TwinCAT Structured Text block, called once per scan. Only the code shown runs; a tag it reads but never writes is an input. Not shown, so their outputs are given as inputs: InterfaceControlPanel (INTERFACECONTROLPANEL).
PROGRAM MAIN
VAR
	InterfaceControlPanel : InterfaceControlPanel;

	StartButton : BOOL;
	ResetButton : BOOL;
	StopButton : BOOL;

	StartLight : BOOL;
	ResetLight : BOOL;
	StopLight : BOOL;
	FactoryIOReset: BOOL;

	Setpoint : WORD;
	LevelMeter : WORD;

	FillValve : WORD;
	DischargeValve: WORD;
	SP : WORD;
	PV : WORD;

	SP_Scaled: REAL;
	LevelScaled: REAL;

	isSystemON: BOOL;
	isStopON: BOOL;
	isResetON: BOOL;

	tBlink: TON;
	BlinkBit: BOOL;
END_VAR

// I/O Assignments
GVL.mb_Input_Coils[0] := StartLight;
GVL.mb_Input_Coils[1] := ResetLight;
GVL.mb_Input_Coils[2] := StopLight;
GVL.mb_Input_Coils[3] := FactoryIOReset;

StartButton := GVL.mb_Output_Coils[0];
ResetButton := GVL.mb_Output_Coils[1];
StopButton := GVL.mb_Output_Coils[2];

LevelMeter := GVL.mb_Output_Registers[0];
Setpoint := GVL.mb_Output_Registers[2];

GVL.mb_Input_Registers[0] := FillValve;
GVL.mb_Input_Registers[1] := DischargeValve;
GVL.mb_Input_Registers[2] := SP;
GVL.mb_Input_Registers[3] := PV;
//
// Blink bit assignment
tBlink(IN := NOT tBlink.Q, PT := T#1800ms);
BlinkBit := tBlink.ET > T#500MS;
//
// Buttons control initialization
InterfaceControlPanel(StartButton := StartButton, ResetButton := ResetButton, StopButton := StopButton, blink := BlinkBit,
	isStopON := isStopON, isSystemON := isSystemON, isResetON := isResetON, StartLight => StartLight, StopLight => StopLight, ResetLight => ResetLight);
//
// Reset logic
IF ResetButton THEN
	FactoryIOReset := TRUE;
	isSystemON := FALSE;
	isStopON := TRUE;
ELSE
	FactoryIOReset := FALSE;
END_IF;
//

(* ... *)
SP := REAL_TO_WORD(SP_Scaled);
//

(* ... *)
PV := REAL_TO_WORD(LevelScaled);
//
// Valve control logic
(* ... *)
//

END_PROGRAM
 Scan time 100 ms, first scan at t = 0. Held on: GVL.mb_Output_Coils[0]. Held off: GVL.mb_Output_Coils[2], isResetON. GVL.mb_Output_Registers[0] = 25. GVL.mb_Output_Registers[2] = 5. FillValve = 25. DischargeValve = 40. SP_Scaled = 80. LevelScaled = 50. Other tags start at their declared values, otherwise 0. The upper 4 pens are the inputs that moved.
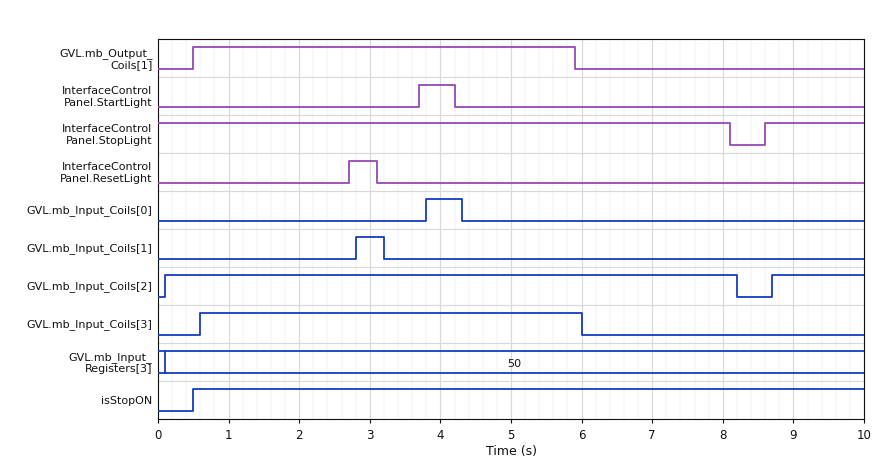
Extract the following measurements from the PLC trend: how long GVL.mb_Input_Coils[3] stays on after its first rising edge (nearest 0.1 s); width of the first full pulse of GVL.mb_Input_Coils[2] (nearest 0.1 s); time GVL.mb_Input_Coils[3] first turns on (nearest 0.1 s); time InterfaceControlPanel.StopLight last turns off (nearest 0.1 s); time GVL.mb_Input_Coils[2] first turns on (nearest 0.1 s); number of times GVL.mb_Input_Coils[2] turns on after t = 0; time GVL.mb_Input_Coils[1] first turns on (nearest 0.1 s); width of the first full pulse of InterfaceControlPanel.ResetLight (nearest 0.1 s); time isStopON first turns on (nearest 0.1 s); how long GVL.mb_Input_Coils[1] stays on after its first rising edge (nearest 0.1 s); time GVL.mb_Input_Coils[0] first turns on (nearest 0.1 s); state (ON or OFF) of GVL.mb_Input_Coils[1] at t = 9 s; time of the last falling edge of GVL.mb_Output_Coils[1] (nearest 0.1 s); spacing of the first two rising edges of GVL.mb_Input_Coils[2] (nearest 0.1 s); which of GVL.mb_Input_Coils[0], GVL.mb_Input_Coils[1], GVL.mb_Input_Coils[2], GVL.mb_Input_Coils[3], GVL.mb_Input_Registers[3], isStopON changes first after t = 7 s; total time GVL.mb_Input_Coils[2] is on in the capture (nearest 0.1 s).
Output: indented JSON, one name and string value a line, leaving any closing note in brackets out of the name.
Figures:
{
  "how long GVL.mb_Input_Coils[3] stays on after its first rising edge": "5.4 s",
  "width of the first full pulse of GVL.mb_Input_Coils[2]": "8.1 s",
  "time GVL.mb_Input_Coils[3] first turns on": "0.6 s",
  "time InterfaceControlPanel.StopLight last turns off": "8.1 s",
  "time GVL.mb_Input_Coils[2] first turns on": "0.1 s",
  "number of times GVL.mb_Input_Coils[2] turns on after t = 0": "2",
  "time GVL.mb_Input_Coils[1] first turns on": "2.8 s",
  "width of the first full pulse of InterfaceControlPanel.ResetLight": "0.4 s",
  "time isStopON first turns on": "0.5 s",
  "how long GVL.mb_Input_Coils[1] stays on after its first rising edge": "0.4 s",
  "time GVL.mb_Input_Coils[0] first turns on": "3.8 s",
  "state (ON or OFF) of GVL.mb_Input_Coils[1] at t = 9 s": "OFF",
  "time of the last falling edge of GVL.mb_Output_Coils[1]": "5.9 s",
  "spacing of the first two rising edges of GVL.mb_Input_Coils[2]": "8.6 s",
  "which of GVL.mb_Input_Coils[0], GVL.mb_Input_Coils[1], GVL.mb_Input_Coils[2], GVL.mb_Input_Coils[3], GVL.mb_Input_Registers[3], isStopON changes first after t = 7 s": "GVL.mb_Input_Coils[2]",
  "total time GVL.mb_Input_Coils[2] is on in the capture": "9.4 s"
}
